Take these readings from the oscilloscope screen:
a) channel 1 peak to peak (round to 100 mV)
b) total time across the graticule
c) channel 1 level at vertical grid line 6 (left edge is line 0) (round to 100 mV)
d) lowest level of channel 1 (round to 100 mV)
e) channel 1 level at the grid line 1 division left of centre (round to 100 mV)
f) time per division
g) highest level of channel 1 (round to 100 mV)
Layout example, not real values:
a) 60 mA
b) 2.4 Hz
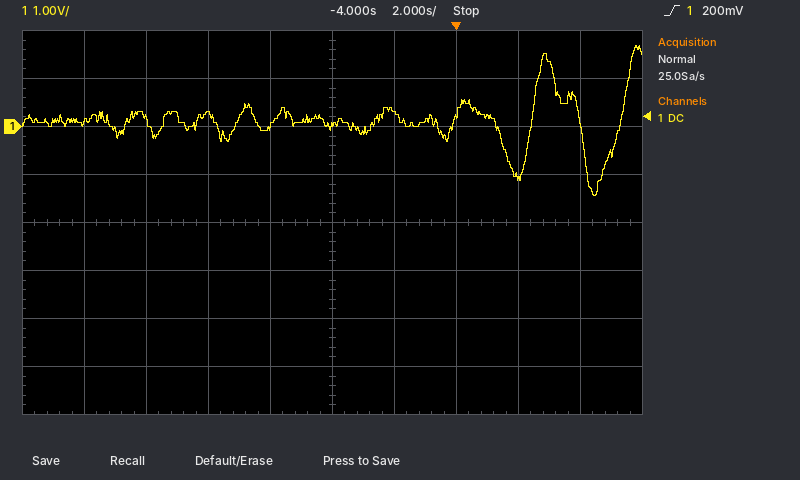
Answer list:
a) 3.1 V
b) 20 s
c) 300 mV
d) -1.4 V
e) 0.0 V
f) 2 s
g) 1.7 V
